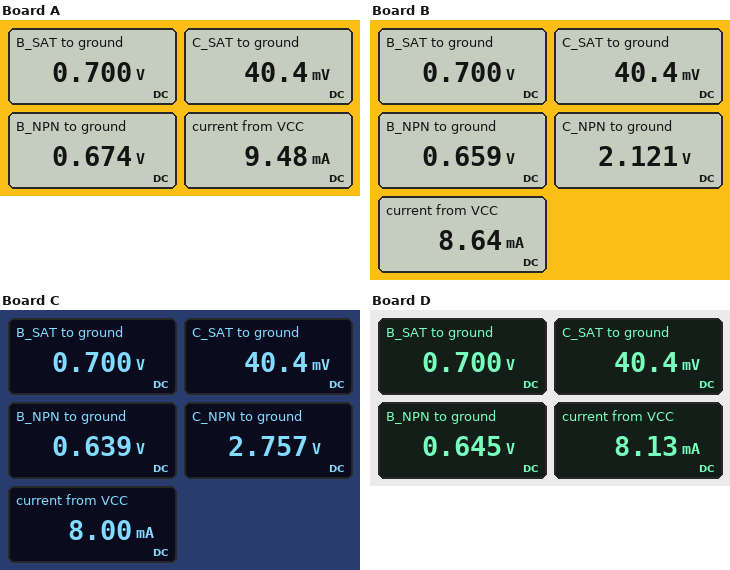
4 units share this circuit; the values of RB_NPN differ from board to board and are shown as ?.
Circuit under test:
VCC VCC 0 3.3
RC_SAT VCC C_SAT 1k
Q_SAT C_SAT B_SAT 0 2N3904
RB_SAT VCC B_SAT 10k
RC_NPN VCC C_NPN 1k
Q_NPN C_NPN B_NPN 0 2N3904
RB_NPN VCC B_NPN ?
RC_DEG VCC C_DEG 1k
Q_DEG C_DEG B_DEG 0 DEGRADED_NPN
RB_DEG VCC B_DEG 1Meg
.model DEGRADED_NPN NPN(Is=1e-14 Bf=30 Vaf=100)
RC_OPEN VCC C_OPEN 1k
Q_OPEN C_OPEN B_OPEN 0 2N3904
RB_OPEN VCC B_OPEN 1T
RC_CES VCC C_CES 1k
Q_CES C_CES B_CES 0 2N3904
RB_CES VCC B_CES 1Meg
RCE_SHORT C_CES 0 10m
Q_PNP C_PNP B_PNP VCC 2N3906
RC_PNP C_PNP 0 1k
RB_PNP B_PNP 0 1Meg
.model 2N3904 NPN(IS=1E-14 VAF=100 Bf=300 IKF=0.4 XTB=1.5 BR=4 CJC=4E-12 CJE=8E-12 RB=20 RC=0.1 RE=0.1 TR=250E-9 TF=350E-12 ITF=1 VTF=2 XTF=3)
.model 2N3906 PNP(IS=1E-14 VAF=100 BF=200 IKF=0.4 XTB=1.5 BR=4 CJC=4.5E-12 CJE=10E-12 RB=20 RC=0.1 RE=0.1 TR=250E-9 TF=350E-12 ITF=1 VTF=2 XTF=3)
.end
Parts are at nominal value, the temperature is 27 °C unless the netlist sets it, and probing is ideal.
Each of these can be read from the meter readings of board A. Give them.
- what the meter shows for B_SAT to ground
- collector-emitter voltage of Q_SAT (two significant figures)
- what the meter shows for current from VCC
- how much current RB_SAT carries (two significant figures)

0.700 V
40 mV
9.48 mA
260 µA
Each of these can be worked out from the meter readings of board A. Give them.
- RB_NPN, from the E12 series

390 kΩ
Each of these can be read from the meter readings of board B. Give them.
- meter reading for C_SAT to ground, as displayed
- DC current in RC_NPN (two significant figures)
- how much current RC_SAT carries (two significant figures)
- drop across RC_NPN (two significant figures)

40.4 mV
1.2 mA
3.3 mA
1.2 V
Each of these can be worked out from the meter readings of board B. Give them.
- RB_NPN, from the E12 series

680 kΩ
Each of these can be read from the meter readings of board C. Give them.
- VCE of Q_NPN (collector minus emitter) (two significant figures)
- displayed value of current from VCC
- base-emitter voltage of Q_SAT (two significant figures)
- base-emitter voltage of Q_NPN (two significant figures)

2.8 V
8.00 mA
700 mV
640 mV
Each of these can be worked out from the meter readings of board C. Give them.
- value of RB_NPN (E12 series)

1.5 MΩ
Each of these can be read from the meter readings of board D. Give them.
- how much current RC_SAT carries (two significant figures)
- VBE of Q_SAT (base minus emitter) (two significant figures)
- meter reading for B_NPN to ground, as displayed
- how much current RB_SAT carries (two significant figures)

3.3 mA
700 mV
0.645 V
260 µA
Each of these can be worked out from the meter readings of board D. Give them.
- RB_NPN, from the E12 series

1.2 MΩ
